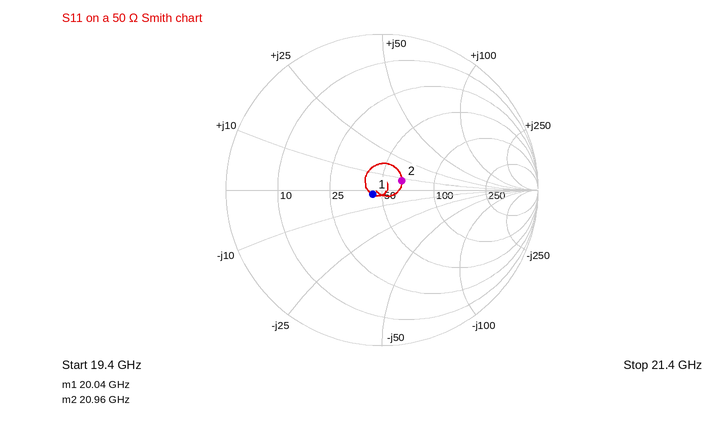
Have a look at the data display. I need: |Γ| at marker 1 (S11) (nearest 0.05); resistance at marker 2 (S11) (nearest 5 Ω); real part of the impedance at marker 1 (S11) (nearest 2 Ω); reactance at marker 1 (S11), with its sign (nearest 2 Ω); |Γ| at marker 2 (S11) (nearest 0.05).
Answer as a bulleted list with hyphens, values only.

- 0.05
- 65 Ω
- 44 Ω
- -2 Ω
- 0.15
